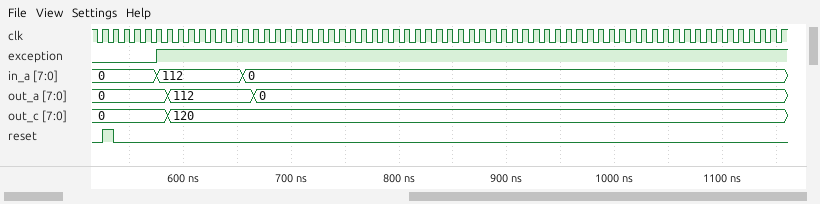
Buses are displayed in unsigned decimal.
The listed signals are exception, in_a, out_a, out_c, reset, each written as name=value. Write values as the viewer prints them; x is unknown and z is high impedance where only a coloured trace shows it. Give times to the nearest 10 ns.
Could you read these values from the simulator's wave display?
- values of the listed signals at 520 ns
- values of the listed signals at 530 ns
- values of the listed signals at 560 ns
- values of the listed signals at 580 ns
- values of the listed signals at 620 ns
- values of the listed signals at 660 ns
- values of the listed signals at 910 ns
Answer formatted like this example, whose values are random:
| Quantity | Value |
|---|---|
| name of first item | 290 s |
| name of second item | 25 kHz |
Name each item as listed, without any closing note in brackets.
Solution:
| Quantity | Value |
|---|---|
| values of the listed signals at 520 ns | exception=0, in_a=0, out_a=0, out_c=0, reset=0 |
| values of the listed signals at 530 ns | exception=0, in_a=0, out_a=0, out_c=0, reset=1 |
| values of the listed signals at 560 ns | exception=0, in_a=0, out_a=0, out_c=0, reset=0 |
| values of the listed signals at 580 ns | exception=1, in_a=112, out_a=0, out_c=0, reset=0 |
| values of the listed signals at 620 ns | exception=1, in_a=112, out_a=112, out_c=120, reset=0 |
| values of the listed signals at 660 ns | exception=1, in_a=0, out_a=112, out_c=120, reset=0 |
| values of the listed signals at 910 ns | exception=1, in_a=0, out_a=0, out_c=120, reset=0 |
